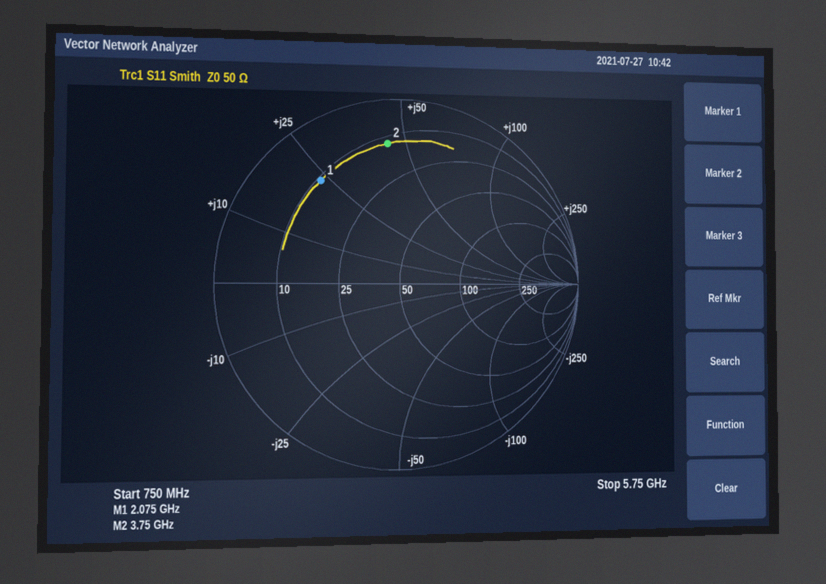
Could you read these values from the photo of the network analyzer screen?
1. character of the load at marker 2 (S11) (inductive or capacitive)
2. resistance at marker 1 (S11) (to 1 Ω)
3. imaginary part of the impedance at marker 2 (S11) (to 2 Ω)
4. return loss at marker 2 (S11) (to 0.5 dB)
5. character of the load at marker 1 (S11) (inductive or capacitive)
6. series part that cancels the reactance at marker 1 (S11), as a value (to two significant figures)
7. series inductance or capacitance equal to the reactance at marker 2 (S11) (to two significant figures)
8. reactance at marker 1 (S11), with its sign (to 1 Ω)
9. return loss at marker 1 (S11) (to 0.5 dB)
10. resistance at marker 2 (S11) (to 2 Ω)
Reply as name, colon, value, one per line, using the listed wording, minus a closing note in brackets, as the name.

character of the load at marker 2 (S11): inductive
resistance at marker 1 (S11): 11 Ω
imaginary part of the impedance at marker 2 (S11): +44 Ω
return loss at marker 2 (S11): 2.5 dB
character of the load at marker 1 (S11): inductive
series part that cancels the reactance at marker 1 (S11), as a value: 3.3 pF
series inductance or capacitance equal to the reactance at marker 2 (S11): 1.9 nH
reactance at marker 1 (S11), with its sign: +23 Ω
return loss at marker 1 (S11): 3.0 dB
resistance at marker 2 (S11): 12 Ω
